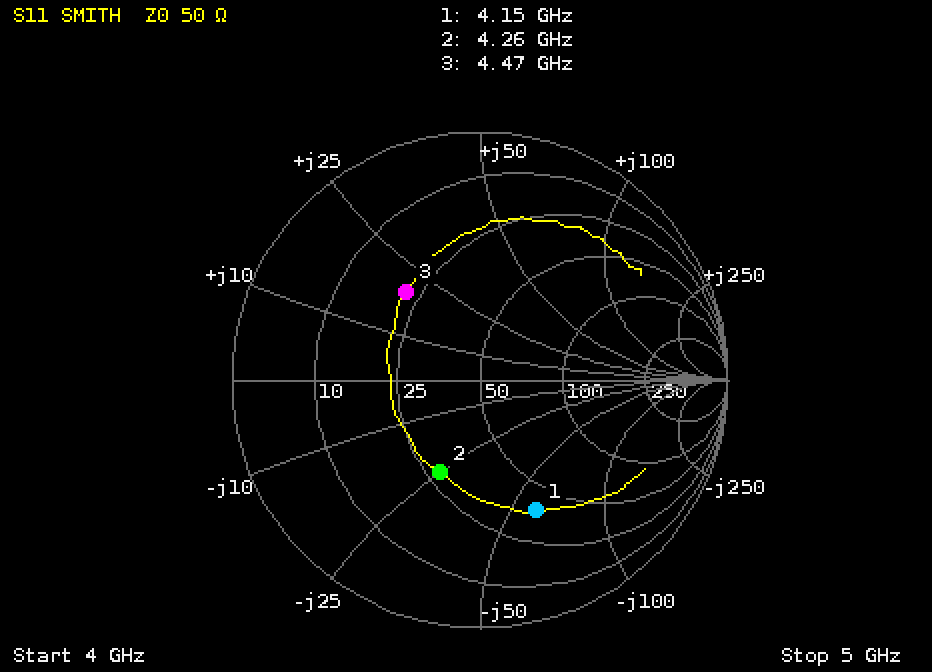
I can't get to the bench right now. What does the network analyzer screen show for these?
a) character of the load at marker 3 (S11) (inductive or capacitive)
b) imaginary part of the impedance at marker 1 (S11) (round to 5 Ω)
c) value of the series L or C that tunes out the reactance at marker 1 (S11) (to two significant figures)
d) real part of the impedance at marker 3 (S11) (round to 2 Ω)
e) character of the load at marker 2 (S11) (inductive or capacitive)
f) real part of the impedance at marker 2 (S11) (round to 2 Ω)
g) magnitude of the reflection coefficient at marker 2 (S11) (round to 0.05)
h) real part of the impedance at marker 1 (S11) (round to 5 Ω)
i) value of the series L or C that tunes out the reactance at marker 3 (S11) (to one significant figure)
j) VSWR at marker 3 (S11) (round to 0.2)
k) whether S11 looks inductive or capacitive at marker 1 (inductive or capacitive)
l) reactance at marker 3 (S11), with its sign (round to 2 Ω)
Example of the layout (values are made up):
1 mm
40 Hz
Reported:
inductive
-60 Ω
2.3 nH
22 Ω
capacitive
28 Ω
0.40
40 Ω
2 pF
2.8
capacitive
+20 Ω
